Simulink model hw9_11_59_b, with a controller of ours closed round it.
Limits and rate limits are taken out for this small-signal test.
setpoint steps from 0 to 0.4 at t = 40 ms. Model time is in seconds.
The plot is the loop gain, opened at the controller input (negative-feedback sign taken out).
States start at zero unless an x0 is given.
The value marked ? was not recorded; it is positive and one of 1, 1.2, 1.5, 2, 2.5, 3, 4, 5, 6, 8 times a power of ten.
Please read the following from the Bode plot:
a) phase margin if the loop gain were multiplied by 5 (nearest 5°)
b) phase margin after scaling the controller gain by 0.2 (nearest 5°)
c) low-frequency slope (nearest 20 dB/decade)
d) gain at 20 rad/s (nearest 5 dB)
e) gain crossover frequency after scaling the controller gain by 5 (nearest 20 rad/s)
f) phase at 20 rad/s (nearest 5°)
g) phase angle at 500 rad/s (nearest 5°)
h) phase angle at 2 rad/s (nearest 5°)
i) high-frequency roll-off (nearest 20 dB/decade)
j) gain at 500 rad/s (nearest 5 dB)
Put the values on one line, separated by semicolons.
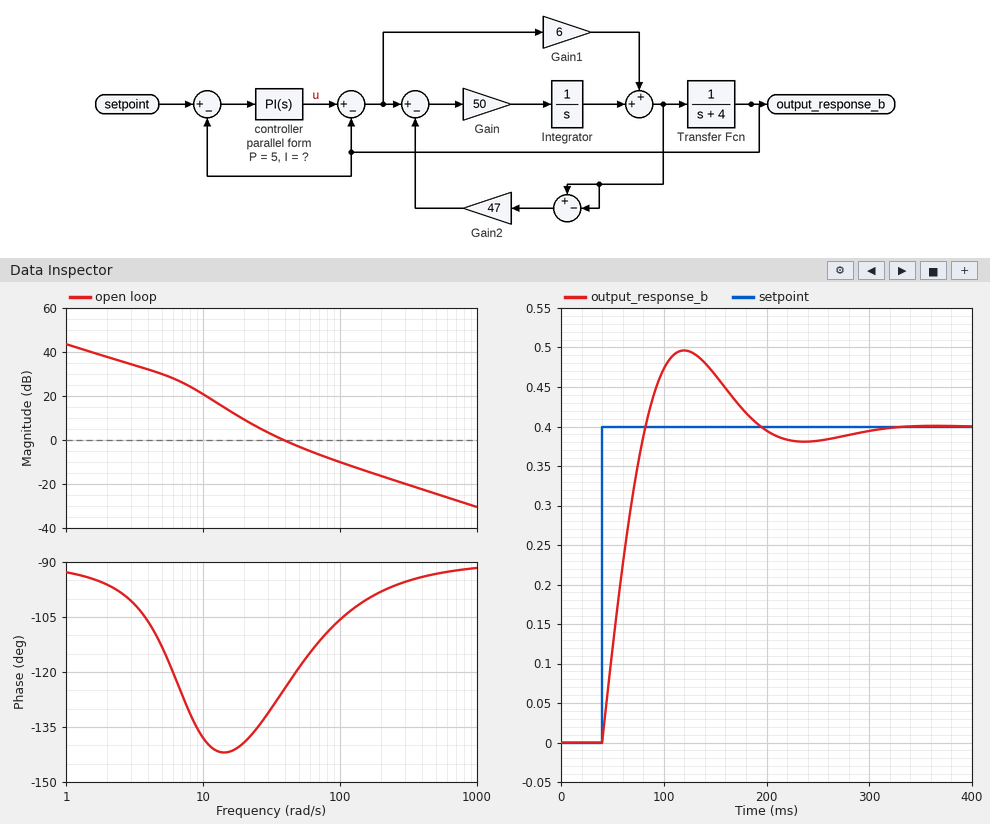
80°; 40°; -20 dB/decade; 10 dB; 160 rad/s; -140°; -95°; -95°; -20 dB/decade; -25 dB
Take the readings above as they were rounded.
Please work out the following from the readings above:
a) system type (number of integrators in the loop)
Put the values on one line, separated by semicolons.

1
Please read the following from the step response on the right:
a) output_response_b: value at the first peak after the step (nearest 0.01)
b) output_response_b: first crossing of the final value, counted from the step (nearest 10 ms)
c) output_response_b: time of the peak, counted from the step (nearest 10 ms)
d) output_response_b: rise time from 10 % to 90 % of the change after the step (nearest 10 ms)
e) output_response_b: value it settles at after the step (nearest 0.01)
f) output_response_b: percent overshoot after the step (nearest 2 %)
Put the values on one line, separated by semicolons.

0.50; 40 ms; 80 ms; 30 ms; 0.40; 24 %
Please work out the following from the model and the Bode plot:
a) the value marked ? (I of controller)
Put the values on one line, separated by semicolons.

150
